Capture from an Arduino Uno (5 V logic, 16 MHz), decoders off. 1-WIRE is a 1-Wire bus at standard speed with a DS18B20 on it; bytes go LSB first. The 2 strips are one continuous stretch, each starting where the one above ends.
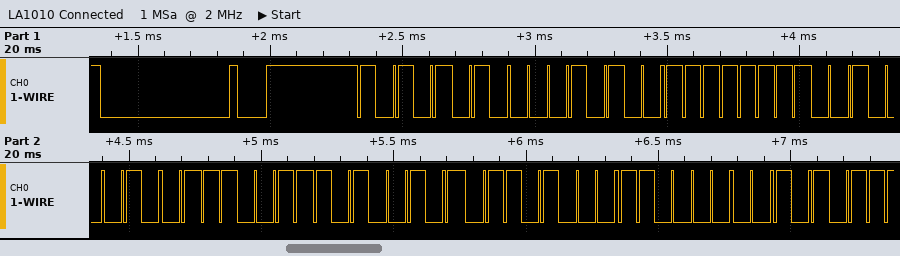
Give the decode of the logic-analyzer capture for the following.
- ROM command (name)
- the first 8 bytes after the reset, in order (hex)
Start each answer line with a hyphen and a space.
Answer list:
- Match ROM
- 55 28 FF 44 CE A5 16 03
